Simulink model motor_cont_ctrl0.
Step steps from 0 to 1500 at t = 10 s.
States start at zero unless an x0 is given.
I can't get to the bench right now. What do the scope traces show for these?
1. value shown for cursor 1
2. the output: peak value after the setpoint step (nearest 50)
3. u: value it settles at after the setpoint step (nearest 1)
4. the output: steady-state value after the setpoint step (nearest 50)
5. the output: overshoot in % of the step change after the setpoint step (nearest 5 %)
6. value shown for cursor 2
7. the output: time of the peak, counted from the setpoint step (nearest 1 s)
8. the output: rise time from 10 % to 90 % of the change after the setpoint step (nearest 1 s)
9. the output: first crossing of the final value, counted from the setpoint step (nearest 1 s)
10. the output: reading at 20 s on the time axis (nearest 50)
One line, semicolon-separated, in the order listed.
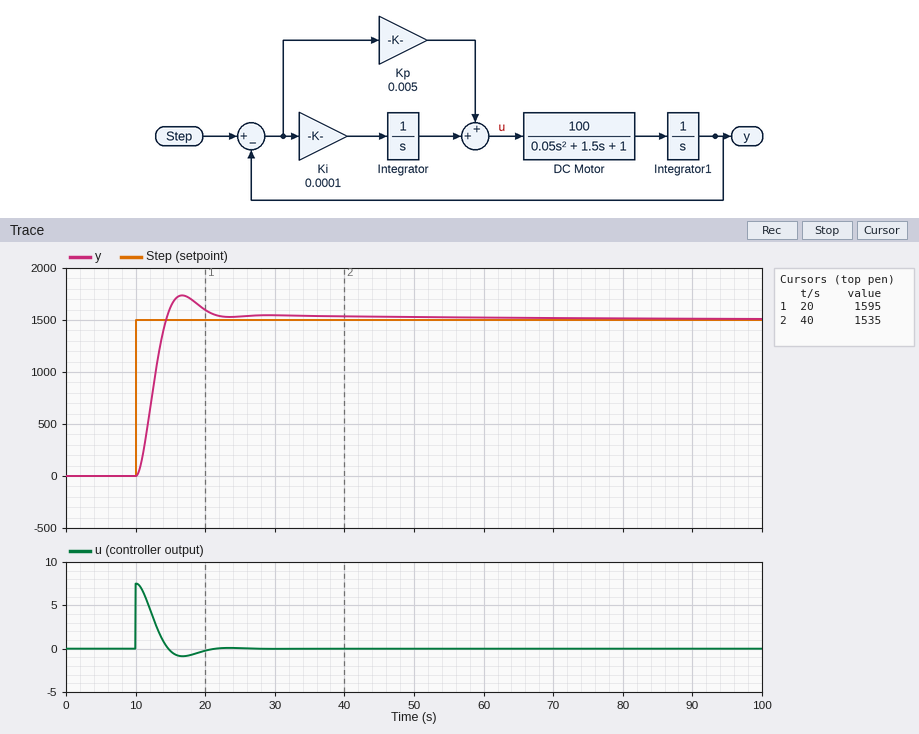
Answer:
1595; 1750; 0; 1500; 15 %; 1535; 7 s; 3 s; 4 s; 1600
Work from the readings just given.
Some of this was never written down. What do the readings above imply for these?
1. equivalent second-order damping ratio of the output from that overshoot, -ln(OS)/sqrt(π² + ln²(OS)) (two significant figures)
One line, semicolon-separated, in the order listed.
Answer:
0.52
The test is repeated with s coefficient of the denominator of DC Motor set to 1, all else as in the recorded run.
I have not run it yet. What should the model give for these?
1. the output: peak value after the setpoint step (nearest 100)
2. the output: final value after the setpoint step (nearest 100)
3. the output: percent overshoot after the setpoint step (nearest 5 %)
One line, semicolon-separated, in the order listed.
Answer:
1600; 1500; 10 %
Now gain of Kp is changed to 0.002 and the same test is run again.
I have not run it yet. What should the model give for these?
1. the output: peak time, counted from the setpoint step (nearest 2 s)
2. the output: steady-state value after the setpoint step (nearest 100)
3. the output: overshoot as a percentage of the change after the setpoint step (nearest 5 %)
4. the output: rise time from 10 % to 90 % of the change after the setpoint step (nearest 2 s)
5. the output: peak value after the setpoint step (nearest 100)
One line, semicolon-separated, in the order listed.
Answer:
16 s; 1500; 20 %; 6 s; 1800
